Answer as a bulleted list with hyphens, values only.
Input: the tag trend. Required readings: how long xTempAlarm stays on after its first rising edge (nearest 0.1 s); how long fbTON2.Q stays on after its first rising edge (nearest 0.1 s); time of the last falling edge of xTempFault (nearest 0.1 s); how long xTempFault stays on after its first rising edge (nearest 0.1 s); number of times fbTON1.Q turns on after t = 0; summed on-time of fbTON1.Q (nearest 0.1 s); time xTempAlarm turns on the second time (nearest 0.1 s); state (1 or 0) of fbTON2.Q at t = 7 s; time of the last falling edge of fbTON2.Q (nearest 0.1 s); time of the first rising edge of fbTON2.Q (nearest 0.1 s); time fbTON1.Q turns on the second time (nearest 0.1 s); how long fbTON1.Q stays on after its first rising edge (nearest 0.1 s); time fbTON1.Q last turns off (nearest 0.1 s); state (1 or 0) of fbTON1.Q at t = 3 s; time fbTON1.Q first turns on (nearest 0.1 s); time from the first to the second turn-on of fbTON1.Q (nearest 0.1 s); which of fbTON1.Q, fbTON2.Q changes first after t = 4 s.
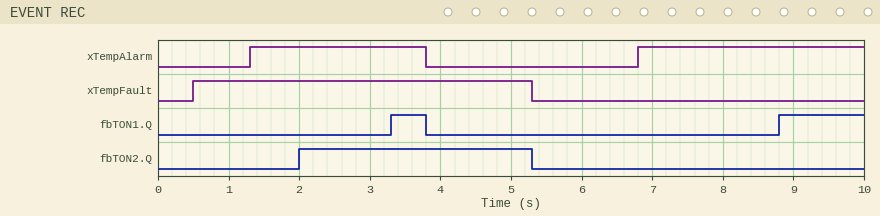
- 2.5 s
- 3.3 s
- 5.3 s
- 4.8 s
- 2
- 1.7 s
- 6.8 s
- 0
- 5.3 s
- 2.0 s
- 8.8 s
- 0.5 s
- 3.8 s
- 0
- 3.3 s
- 5.5 s
- fbTON2.Q
